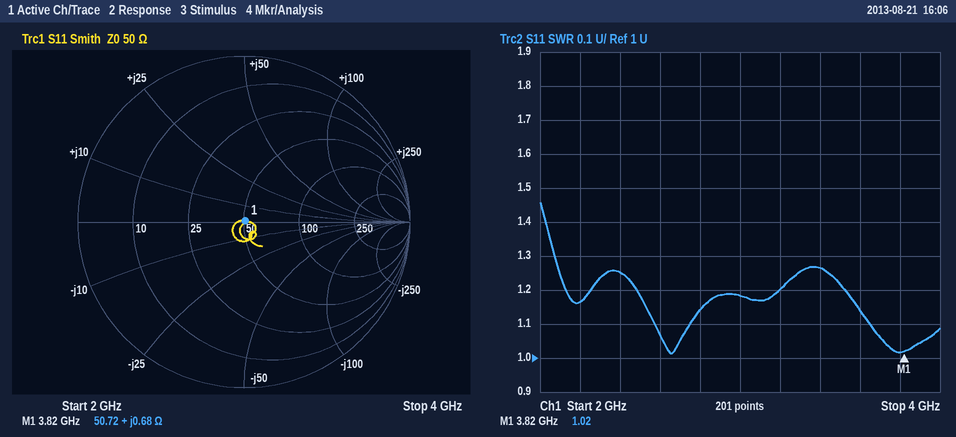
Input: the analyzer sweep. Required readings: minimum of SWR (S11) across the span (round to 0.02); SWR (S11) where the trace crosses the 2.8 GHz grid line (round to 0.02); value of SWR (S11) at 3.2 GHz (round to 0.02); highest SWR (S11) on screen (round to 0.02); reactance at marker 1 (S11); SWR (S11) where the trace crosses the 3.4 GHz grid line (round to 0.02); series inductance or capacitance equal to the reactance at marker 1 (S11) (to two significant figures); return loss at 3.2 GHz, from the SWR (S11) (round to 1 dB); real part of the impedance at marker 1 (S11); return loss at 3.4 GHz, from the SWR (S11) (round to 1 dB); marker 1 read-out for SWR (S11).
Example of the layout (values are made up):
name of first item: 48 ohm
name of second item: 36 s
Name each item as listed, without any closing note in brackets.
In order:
minimum of SWR (S11) across the span: 1.02
SWR (S11) where the trace crosses the 2.8 GHz grid line: 1.14
value of SWR (S11) at 3.2 GHz: 1.20
highest SWR (S11) on screen: 1.46
reactance at marker 1: +0.68 Ω
SWR (S11) where the trace crosses the 3.4 GHz grid line: 1.26
series inductance or capacitance equal to the reactance at marker 1 (S11): 28 pH
return loss at 3.2 GHz, from the SWR (S11): 21 dB
real part of the impedance at marker 1: 50.72 Ω
return loss at 3.4 GHz, from the SWR (S11): 19 dB
marker 1 read-out for SWR: 1.02
